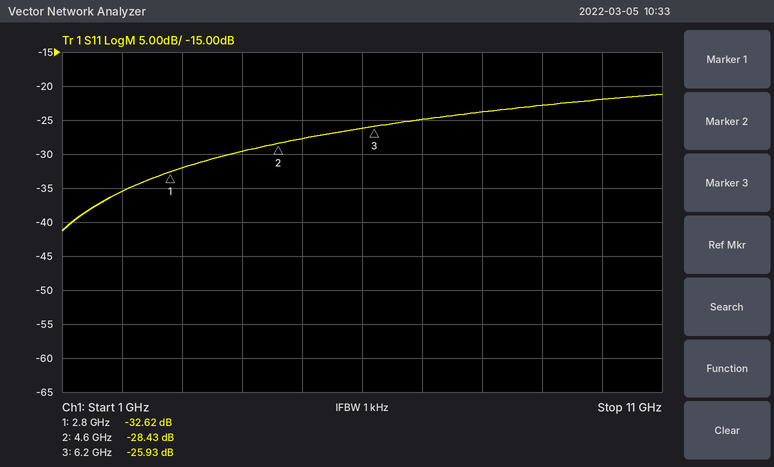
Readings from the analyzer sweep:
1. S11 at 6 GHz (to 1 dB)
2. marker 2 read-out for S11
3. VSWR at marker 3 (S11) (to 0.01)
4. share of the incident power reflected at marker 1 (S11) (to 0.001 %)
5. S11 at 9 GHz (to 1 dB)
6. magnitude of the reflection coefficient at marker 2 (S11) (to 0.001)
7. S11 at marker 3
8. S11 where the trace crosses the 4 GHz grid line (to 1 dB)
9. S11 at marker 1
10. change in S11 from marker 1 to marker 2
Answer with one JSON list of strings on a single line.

["-26 dB", "-28.43 dB", "1.11", "0.055 %", "-23 dB", "0.038", "-25.93 dB", "-30 dB", "-32.62 dB", "4.19 dB"]
